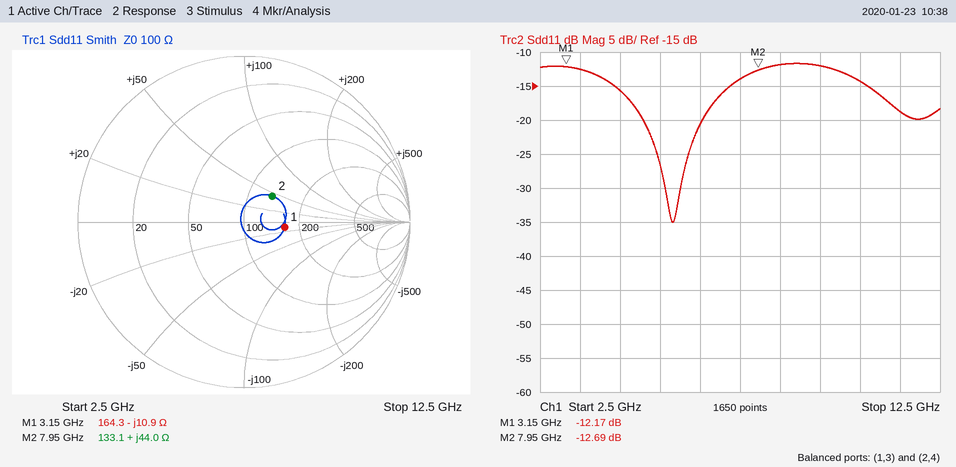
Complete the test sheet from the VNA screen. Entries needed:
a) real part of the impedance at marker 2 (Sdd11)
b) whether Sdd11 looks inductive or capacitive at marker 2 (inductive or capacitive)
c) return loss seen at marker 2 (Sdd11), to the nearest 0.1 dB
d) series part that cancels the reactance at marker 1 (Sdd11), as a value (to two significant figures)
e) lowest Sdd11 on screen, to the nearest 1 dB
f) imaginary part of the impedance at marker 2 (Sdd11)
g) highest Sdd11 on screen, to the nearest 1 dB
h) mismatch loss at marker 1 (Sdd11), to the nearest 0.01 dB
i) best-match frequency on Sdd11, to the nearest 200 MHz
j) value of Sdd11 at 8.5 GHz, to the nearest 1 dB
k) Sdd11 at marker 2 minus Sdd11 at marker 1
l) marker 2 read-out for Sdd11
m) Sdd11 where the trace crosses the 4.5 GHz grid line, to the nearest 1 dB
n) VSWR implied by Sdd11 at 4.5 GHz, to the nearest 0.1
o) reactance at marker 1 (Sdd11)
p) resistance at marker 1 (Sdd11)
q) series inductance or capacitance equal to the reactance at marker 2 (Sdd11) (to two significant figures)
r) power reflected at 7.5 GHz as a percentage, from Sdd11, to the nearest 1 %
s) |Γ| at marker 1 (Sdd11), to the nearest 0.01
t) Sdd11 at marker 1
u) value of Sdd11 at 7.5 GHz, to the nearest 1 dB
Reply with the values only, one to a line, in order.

133.1 Ω
inductive
12.7 dB
550 pH
-35 dB
+44.0 Ω
-12 dB
0.27 dB
5.8 GHz
-12 dB
-0.52 dB
-12.69 dB
-16 dB
1.4
-10.9 Ω
164.3 Ω
880 pH
4 %
0.25
-12.17 dB
-14 dB
